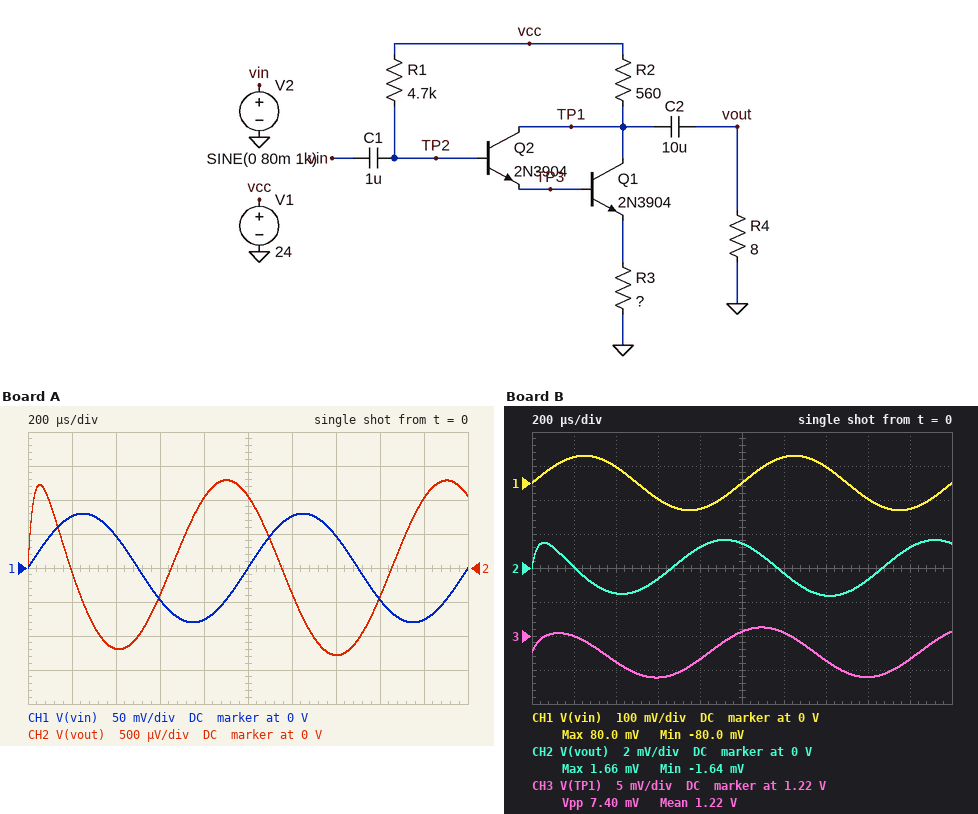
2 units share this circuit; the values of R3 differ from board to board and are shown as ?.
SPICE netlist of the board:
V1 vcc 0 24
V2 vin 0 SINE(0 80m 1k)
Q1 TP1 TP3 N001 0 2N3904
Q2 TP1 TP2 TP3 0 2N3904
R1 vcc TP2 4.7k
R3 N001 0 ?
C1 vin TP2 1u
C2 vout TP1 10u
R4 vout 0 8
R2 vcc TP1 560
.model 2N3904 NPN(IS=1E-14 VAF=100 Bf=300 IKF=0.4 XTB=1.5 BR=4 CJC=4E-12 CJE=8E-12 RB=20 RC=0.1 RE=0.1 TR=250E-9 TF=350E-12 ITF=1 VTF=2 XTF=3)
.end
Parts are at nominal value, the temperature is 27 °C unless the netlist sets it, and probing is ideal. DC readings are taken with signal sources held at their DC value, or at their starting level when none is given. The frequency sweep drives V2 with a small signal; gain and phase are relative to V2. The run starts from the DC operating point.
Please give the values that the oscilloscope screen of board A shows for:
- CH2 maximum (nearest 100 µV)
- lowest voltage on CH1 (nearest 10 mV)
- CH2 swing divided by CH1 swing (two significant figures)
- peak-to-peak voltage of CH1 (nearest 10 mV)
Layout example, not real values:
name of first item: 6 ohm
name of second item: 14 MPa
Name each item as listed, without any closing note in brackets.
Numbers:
CH2 maximum: 1.3 mV
lowest voltage on CH1: -80 mV
CH2 swing divided by CH1 swing: 0.016
peak-to-peak voltage of CH1: 160 mV
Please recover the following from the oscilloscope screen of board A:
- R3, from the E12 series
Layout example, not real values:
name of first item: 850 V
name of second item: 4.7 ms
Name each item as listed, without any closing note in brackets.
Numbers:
R3, from the E12 series: 6.8 Ω
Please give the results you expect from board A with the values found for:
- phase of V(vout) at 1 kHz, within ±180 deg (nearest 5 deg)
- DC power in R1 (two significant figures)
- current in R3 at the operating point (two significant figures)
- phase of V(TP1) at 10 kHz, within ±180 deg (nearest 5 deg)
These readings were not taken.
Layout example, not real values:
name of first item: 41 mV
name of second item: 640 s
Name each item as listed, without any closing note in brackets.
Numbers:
phase of V(vout) at 1 kHz, within ±180 deg: 125 deg
DC power in R1: 100 mW
current in R3 at the operating point: 46 mA
phase of V(TP1) at 10 kHz, within ±180 deg: 25 deg
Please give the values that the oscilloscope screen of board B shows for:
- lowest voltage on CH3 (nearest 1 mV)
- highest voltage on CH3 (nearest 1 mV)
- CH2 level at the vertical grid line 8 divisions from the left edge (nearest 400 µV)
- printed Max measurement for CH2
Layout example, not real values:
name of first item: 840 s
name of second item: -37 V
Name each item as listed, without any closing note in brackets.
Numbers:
lowest voltage on CH3: 1.214 V
highest voltage on CH3: 1.221 V
CH2 level at the vertical grid line 8 divisions from the left edge: -800 µV
printed Max measurement for CH2: 1.66 mV
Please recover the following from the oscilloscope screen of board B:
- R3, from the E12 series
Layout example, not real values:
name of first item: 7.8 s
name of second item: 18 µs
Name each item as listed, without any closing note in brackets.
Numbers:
R3, from the E12 series: 10 Ω
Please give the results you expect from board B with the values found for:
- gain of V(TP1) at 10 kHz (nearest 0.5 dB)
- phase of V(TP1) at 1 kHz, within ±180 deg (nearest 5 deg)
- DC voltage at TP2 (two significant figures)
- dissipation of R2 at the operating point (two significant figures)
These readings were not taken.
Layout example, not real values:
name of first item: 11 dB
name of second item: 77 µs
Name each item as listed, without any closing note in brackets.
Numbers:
gain of V(TP1) at 10 kHz: -17.5 dB
phase of V(TP1) at 1 kHz, within ±180 deg: 55 deg
DC voltage at TP2: 2.0 V
dissipation of R2 at the operating point: 930 mW
